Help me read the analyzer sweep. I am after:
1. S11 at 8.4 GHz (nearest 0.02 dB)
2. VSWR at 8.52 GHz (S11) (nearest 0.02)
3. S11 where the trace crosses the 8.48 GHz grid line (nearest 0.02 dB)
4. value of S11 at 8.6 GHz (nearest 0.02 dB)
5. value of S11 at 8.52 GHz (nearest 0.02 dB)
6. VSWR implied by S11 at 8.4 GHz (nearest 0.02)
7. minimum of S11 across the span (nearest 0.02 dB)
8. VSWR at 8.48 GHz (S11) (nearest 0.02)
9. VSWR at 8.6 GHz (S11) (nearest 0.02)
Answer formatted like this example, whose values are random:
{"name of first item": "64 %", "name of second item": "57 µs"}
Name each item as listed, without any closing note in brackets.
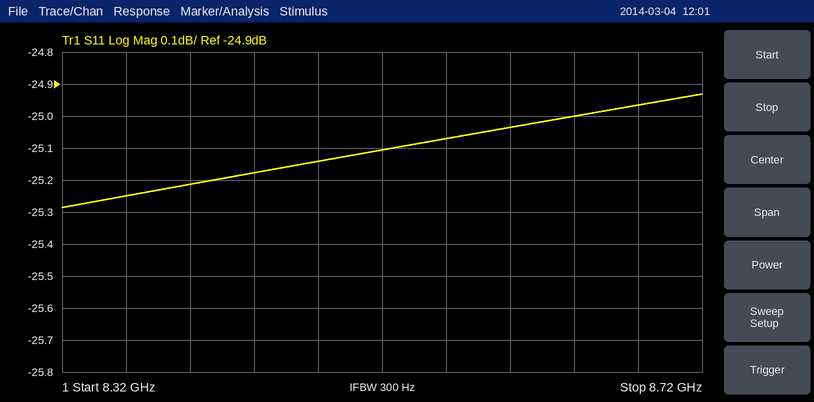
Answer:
{"S11 at 8.4 GHz": "-25.22 dB", "VSWR at 8.52 GHz (S11)": "1.12", "S11 where the trace crosses the 8.48 GHz grid line": "-25.14 dB", "value of S11 at 8.6 GHz": "-25.04 dB", "value of S11 at 8.52 GHz": "-25.10 dB", "VSWR implied by S11 at 8.4 GHz": "1.12", "minimum of S11 across the span": "-25.28 dB", "VSWR at 8.48 GHz (S11)": "1.12", "VSWR at 8.6 GHz (S11)": "1.12"}
